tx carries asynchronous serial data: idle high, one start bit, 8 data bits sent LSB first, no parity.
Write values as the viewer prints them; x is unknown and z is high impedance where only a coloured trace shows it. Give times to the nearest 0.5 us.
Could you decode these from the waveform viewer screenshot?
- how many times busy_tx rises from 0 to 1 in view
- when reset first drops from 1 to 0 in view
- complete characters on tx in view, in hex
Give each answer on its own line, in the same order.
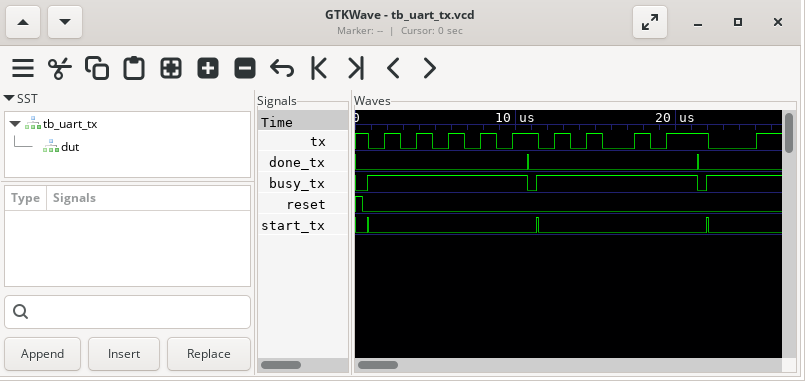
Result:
3
0.5 us
55, A5
